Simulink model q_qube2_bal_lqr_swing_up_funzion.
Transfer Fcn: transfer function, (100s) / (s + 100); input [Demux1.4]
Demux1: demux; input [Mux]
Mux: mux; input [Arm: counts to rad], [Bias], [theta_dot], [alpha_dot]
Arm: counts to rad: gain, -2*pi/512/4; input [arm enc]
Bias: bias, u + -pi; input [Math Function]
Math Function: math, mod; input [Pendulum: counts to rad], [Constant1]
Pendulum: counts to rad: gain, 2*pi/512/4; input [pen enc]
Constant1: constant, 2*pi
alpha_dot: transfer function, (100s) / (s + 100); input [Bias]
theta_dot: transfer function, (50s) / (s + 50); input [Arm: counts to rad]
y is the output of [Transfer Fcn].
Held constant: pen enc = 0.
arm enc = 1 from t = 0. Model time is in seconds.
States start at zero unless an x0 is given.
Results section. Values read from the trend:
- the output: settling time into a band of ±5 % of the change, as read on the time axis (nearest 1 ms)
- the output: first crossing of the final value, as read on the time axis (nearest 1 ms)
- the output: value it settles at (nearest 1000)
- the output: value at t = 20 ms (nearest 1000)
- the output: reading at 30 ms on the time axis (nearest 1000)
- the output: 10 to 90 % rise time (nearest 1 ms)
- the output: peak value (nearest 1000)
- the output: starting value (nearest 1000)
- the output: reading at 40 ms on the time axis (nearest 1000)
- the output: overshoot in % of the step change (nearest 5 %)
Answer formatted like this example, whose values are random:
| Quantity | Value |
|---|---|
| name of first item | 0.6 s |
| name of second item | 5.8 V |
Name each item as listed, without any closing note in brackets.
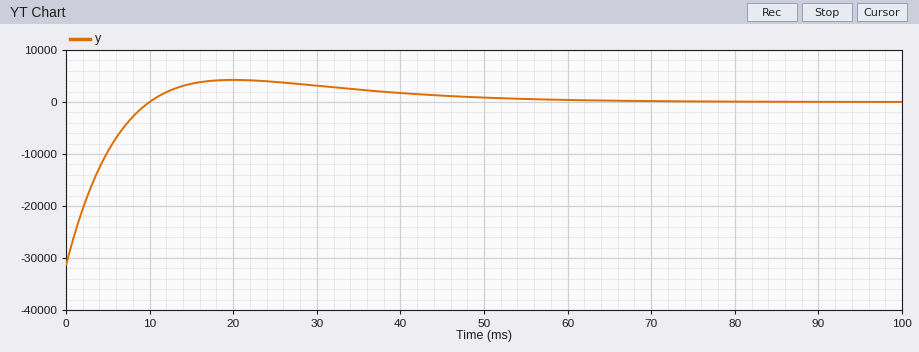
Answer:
| Quantity | Value |
|---|---|
| the output: settling time into a band of ±5 % of the change, as read on the time axis | 41 ms |
| the output: first crossing of the final value, as read on the time axis | 10 ms |
| the output: value it settles at | 0 |
| the output: value at t = 20 ms | 4000 |
| the output: reading at 30 ms on the time axis | 3000 |
| the output: 10 to 90 % rise time | 7 ms |
| the output: peak value | 4000 |
| the output: starting value | -31000 |
| the output: reading at 40 ms on the time axis | 2000 |
| the output: overshoot in % of the step change | 15 % |
